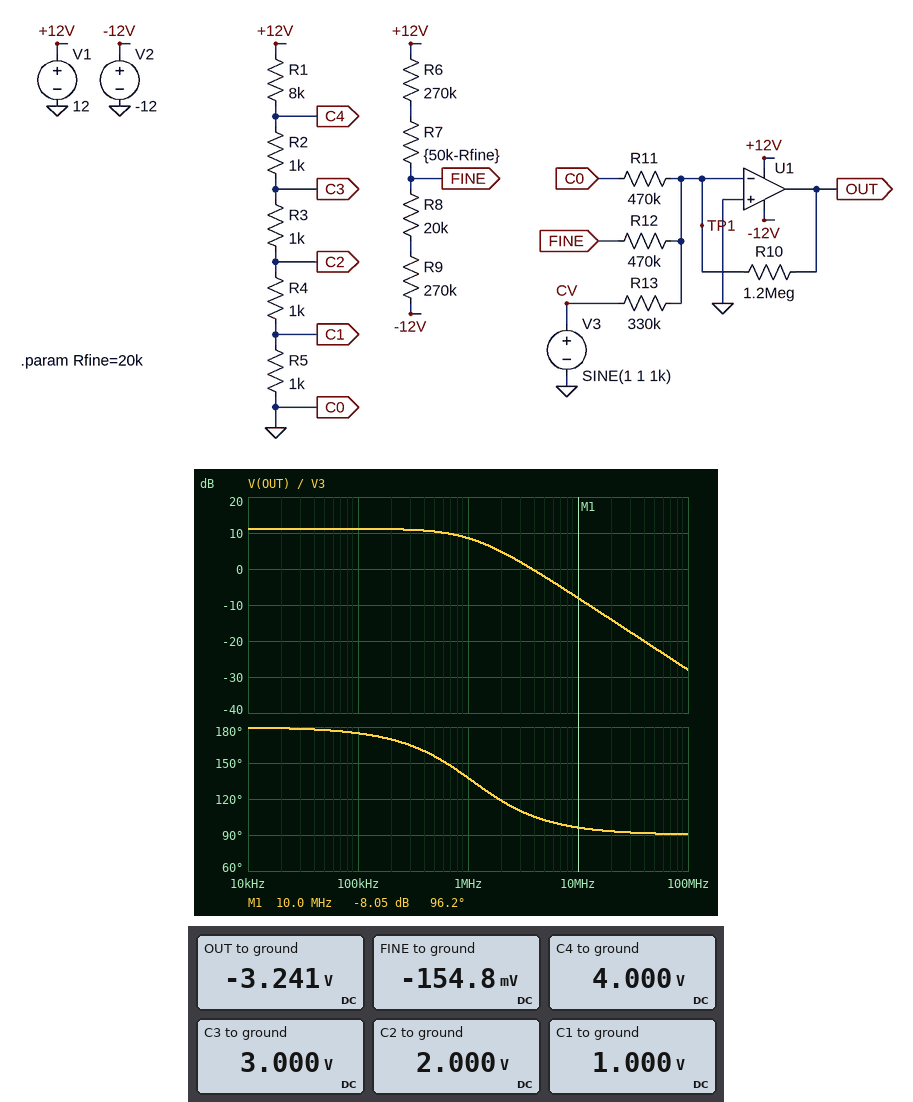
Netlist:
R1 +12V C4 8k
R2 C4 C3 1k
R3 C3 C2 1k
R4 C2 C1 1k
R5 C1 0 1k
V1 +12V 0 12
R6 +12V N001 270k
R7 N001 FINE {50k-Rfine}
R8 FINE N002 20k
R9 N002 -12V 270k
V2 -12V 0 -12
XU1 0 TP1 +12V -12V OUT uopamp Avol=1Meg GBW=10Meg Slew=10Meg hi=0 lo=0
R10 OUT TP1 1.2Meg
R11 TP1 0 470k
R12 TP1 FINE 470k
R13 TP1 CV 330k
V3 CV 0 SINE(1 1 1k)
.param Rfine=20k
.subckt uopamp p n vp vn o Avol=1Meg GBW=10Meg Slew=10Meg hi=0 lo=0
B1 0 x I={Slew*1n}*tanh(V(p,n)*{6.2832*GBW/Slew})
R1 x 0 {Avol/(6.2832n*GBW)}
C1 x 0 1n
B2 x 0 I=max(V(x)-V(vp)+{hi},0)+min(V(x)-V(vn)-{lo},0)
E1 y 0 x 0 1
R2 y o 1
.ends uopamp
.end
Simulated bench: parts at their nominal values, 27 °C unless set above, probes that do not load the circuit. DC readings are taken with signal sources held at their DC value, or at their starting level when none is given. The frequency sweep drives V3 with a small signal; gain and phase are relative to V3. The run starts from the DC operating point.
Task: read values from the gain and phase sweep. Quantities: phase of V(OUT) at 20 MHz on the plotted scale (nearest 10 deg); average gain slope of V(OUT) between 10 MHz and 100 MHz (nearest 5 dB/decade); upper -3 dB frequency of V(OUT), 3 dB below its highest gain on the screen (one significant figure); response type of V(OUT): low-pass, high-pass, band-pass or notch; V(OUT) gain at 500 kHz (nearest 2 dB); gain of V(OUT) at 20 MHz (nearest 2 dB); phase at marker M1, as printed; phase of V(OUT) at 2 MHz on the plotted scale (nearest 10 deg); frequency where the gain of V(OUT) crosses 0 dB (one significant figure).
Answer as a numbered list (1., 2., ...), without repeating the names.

1. 90 deg
2. -20 dB/decade
3. 1 MHz
4. low-pass
5. 10 dB
6. -14 dB
7. 96.2 deg
8. 120 deg
9. 4 MHz
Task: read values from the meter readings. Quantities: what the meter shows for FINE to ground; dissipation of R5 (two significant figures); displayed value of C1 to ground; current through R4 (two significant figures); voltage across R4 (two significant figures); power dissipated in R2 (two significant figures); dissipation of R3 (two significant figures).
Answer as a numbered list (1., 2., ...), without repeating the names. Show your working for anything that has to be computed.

1. -154.8 mV
2. (1 V)^2 / 1 kΩ = 1.0 mW
3. 1.000 V
4. (2 V - 1 V) / 1 kΩ = 1.0 mA
5. 2 V - 1 V = 1.0 V
6. (4 V - 3 V)^2 / 1 kΩ = 1.0 mW
7. (3 V - 2 V)^2 / 1 kΩ = 1.0 mW
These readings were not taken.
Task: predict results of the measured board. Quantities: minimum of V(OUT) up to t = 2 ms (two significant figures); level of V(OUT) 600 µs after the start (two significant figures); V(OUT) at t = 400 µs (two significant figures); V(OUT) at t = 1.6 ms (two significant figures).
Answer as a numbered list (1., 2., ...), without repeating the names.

1. -6.9 V
2. -1.1 V
3. -5.4 V
4. -1.1 V
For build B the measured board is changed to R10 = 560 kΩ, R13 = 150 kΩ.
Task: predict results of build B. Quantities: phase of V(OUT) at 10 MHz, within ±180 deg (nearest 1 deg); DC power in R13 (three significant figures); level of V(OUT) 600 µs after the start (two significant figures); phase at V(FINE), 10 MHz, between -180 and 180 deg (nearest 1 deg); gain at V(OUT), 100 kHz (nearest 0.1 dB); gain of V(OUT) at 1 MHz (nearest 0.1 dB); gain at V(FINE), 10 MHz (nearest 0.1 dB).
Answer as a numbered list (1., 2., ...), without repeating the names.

1. 98 deg
2. 6.67 µW
3. -1.4 V
4. 8 deg
5. 11.4 dB
6. 9.8 dB
7. -17.8 dB
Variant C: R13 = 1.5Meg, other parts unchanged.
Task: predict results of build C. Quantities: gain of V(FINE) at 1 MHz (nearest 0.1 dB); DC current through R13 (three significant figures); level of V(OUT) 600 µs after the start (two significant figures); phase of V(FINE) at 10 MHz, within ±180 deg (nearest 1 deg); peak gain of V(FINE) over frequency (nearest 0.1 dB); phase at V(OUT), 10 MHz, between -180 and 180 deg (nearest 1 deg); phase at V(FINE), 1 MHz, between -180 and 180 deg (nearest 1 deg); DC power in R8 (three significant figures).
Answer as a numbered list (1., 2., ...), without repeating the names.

1. -35.8 dB
2. 667 nA
3. 65 mV
4. 9 deg
5. -30.4 dB
6. 99 deg
7. 58 deg
8. 33.4 µW
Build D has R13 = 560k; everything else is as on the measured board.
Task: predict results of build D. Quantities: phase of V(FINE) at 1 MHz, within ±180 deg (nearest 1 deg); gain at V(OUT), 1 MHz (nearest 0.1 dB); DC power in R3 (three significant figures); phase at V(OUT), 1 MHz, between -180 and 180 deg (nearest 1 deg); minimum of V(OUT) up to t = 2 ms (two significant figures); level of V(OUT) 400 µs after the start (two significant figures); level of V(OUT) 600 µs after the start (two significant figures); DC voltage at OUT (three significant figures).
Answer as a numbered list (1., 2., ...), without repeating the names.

1. 53 deg
2. 4.6 dB
3. 1.00 mW
4. 143 deg
5. -3.9 V
6. -3.0 V
7. -490 mV
8. -1.75 V
